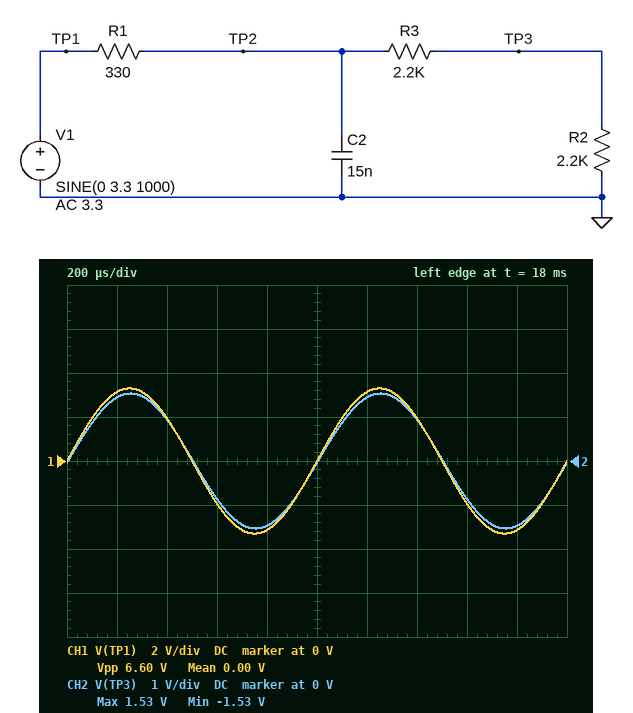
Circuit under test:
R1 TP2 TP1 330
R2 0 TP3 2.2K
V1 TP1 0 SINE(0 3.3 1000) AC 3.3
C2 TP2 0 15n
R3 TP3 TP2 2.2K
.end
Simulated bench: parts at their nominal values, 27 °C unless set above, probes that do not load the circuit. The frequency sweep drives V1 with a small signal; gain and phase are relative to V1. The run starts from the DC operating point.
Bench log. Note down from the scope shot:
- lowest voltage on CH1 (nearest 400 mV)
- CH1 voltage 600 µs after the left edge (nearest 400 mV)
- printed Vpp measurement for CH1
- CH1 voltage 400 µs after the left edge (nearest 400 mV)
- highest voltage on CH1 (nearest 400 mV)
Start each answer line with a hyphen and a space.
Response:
- -3.2 V
- -2.0 V
- 6.60 V
- 2.0 V
- 3.2 V
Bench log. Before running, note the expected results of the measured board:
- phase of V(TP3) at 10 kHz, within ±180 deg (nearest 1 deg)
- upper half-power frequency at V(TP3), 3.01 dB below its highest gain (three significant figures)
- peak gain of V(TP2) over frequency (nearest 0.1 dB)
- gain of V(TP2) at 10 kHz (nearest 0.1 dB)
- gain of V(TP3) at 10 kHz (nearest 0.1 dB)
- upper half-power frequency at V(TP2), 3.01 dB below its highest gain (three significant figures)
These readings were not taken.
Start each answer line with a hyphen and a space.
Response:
- -16 deg
- 34.6 kHz
- -0.6 dB
- -1.0 dB
- -7.0 dB
- 34.6 kHz
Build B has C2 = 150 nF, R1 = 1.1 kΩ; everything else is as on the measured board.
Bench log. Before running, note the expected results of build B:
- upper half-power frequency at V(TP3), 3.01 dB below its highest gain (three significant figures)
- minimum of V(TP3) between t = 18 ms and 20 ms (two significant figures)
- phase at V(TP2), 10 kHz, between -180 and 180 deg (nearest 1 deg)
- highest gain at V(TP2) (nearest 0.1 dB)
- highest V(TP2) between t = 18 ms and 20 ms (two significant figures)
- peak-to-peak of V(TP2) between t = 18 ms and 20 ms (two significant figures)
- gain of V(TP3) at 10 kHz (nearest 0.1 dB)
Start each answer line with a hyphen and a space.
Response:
- 1.21 kHz
- -1.0 V
- -83 deg
- -1.9 dB
- 2.0 V
- 4.1 V
- -26.4 dB
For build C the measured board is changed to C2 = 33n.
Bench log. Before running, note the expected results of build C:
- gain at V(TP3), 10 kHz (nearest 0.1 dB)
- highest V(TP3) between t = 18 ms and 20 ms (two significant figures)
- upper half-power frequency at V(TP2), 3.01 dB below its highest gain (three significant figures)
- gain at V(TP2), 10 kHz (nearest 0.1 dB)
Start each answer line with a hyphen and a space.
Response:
- -8.1 dB
- 1.5 V
- 15.7 kHz
- -2.1 dB
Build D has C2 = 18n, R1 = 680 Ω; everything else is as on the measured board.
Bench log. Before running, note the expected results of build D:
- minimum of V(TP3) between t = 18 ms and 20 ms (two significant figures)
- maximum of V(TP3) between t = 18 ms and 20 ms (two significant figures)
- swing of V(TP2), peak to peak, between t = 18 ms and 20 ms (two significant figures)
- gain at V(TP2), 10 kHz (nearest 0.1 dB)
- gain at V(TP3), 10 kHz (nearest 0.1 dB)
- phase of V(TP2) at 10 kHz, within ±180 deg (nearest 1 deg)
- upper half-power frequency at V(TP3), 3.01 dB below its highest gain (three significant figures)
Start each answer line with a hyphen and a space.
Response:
- -1.4 V
- 1.4 V
- 5.7 V
- -2.8 dB
- -8.9 dB
- -34 deg
- 15.0 kHz
